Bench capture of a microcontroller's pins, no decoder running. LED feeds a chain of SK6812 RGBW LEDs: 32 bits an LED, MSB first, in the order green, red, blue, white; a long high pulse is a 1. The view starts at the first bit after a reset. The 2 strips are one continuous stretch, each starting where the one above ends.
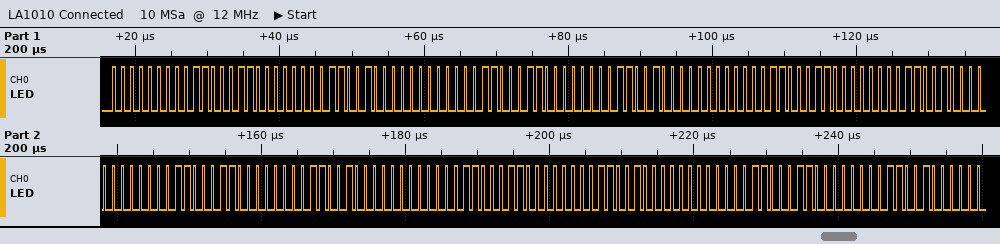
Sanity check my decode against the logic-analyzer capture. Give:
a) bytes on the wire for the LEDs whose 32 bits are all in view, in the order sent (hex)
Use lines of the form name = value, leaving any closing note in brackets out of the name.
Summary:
bytes on the wire for the LEDs whose 32 bits are all in view, in the order sent = 00 63 00 C8 00 63 00 C8 00 63 00 C8 00 63 00 C8 00 63 00 C8 00 63 00 C8
